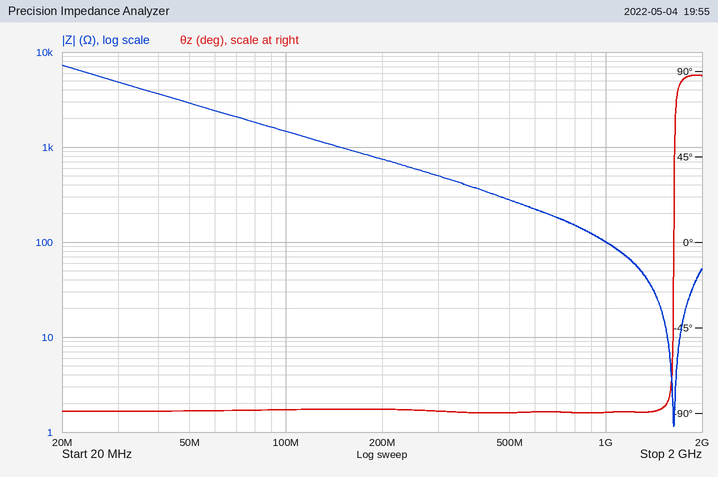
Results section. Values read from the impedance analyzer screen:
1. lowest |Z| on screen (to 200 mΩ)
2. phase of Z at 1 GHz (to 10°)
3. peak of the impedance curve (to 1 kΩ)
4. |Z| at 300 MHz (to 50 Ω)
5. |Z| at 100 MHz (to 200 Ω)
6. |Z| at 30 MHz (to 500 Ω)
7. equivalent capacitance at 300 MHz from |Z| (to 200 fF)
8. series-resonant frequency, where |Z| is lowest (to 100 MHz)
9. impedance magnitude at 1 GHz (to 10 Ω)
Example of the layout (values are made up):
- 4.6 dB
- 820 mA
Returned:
- 1.2 Ω
- -90°
- 7 kΩ
- 500 Ω
- 1.4 kΩ
- 5.0 kΩ
- 1.0 pF
- 1.6 GHz
- 100 Ω
